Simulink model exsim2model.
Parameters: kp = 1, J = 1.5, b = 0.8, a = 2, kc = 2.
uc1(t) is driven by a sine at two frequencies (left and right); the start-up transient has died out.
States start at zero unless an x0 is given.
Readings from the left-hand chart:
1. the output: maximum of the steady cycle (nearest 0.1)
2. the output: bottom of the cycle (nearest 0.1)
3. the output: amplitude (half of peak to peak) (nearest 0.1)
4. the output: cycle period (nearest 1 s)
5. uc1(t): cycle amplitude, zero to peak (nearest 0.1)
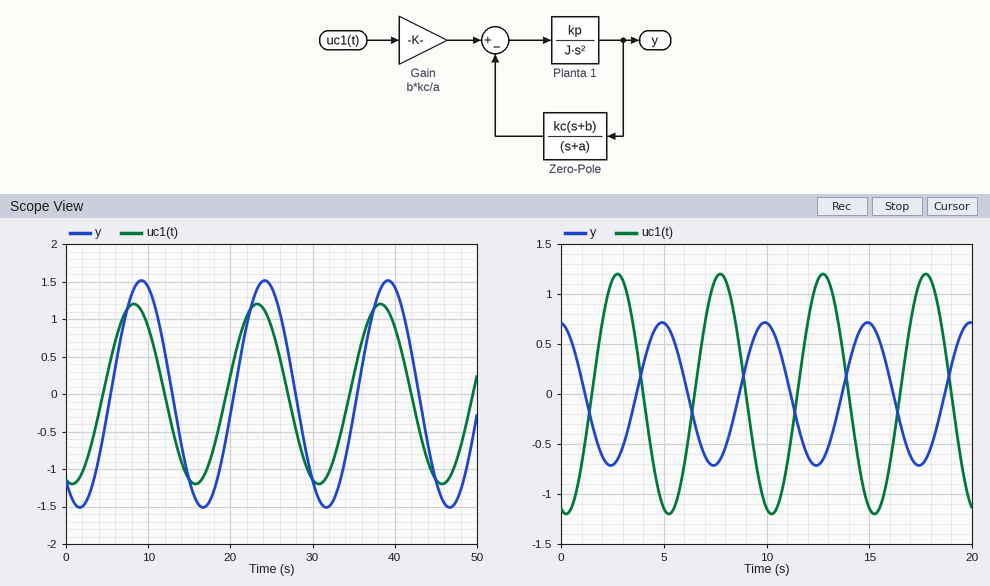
1.5
-1.5
1.5
15 s
1.2
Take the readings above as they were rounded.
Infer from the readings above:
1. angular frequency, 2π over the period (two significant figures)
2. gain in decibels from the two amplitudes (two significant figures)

0.42 rad/s
1.9 dB
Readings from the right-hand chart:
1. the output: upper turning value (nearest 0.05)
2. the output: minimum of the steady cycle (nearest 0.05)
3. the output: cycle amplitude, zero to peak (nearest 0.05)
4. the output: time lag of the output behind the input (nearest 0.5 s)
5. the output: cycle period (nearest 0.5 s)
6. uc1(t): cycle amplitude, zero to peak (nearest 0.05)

0.70
-0.70
0.70
2.0 s
5.0 s
1.20
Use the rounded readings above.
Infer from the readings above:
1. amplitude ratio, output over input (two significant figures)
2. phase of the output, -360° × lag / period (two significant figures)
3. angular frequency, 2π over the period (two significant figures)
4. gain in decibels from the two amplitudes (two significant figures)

0.58
-140°
1.3 rad/s
-4.7 dB
